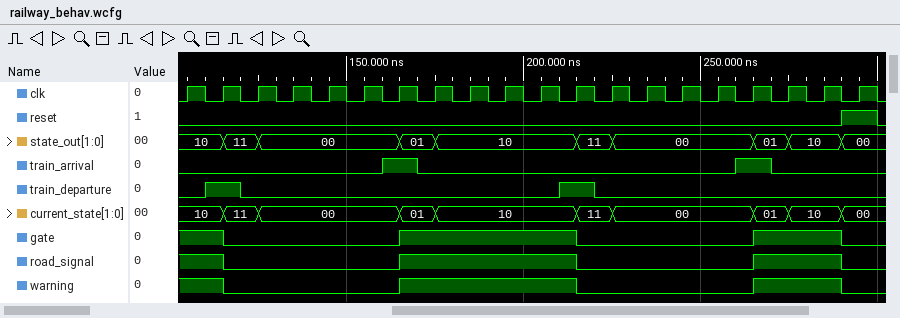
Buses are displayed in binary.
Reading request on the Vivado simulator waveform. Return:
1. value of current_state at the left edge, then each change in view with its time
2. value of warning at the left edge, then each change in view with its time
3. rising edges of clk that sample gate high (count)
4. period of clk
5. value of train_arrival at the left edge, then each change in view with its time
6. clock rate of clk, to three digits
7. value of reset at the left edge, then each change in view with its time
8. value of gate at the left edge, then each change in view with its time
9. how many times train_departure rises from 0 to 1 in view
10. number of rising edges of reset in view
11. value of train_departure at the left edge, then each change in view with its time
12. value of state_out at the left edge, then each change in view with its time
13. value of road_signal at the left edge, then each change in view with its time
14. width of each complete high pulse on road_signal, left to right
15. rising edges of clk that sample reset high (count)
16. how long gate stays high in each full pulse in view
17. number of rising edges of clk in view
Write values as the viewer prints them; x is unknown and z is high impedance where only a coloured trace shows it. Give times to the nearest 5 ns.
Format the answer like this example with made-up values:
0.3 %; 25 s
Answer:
10, 11 at 115 ns, 00 at 125 ns, 01 at 165 ns, 10 at 175 ns, 11 at 215 ns, 00 at 225 ns, 01 at 265 ns, 10 at 275 ns, 00 at 290 ns; 1, 0 at 115 ns, 1 at 165 ns, 0 at 215 ns, 1 at 265 ns, 0 at 290 ns; 9; 10 ns; 0, 1 at 160 ns, 0 at 170 ns, 1 at 260 ns, 0 at 270 ns; 100 MHz; 0, 1 at 290 ns, 0 at 300 ns; 1, 0 at 115 ns, 1 at 165 ns, 0 at 215 ns, 1 at 265 ns, 0 at 290 ns; 2; 1; 0, 1 at 110 ns, 0 at 120 ns, 1 at 210 ns, 0 at 220 ns; 10, 11 at 115 ns, 00 at 125 ns, 01 at 165 ns, 10 at 175 ns, 11 at 215 ns, 00 at 225 ns, 01 at 265 ns, 10 at 275 ns, 00 at 290 ns; 1, 0 at 115 ns, 1 at 165 ns, 0 at 215 ns, 1 at 265 ns, 0 at 290 ns; 50 ns, 25 ns; 1; 50 ns, 25 ns; 20
